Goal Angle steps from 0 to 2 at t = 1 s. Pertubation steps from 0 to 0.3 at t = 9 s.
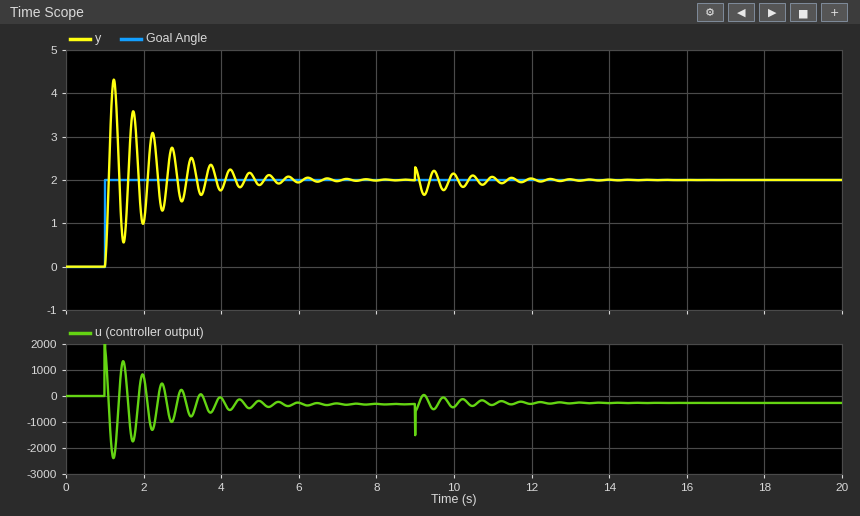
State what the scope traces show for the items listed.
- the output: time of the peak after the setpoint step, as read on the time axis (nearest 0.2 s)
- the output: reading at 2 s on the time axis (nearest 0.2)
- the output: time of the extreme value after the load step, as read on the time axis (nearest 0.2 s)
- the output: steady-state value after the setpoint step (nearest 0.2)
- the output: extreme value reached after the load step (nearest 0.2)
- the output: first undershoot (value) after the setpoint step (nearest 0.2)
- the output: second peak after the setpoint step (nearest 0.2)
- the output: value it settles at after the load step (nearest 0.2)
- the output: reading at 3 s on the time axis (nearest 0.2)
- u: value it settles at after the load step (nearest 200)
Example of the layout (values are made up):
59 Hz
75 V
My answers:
1.2 s
1.0
9.2 s
2.0
1.6
0.6
3.6
2.0
1.6
-200
